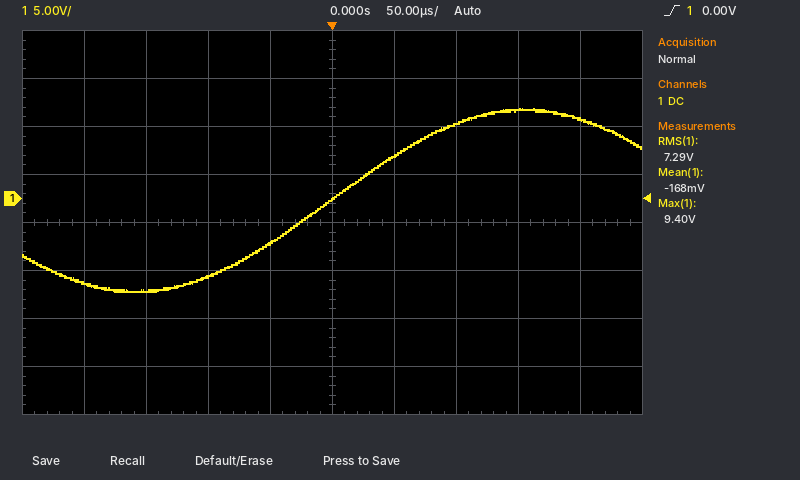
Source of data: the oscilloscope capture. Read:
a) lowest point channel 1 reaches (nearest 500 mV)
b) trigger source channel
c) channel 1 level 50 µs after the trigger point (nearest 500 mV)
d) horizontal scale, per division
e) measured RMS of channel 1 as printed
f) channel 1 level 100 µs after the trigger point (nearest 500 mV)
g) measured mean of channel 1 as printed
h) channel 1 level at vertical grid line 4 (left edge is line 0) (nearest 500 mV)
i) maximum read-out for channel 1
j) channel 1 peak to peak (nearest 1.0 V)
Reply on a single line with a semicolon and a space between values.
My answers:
-9.5 V; channel 1; 4.5 V; 50 µs; 7.29 V; 8.0 V; -168 mV; -4.5 V; 9.40 V; 19.0 V
